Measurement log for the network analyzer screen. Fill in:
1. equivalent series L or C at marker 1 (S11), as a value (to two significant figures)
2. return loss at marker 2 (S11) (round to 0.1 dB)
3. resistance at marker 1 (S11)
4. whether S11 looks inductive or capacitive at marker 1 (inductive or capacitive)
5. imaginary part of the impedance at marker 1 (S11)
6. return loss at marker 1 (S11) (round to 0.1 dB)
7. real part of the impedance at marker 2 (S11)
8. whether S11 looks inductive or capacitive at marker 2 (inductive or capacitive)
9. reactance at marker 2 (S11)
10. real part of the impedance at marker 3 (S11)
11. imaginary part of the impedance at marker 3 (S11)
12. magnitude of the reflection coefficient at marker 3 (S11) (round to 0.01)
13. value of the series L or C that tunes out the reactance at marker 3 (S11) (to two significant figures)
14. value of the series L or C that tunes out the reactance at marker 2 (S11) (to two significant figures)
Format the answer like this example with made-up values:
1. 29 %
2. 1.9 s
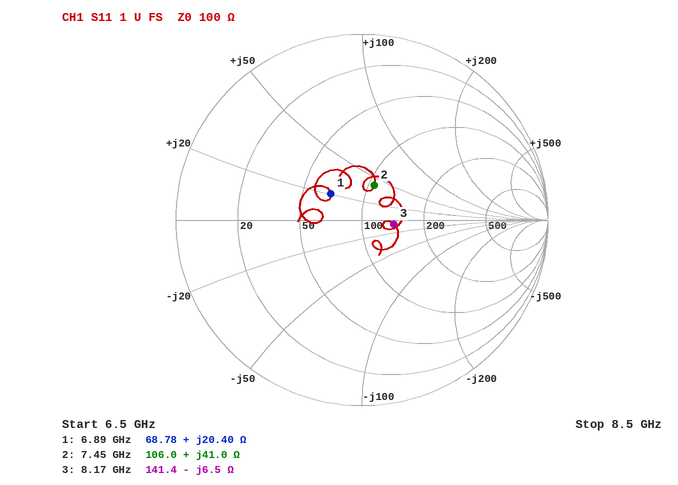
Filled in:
1. 470 pH
2. 14.1 dB
3. 68.78 Ω
4. inductive
5. +20.40 Ω
6. 13.2 dB
7. 106.0 Ω
8. inductive
9. +41.0 Ω
10. 141.4 Ω
11. -6.5 Ω
12. 0.17
13. 130 pH
14. 520 fF
